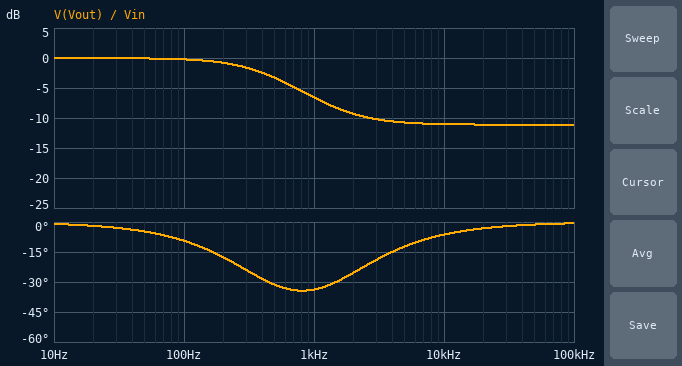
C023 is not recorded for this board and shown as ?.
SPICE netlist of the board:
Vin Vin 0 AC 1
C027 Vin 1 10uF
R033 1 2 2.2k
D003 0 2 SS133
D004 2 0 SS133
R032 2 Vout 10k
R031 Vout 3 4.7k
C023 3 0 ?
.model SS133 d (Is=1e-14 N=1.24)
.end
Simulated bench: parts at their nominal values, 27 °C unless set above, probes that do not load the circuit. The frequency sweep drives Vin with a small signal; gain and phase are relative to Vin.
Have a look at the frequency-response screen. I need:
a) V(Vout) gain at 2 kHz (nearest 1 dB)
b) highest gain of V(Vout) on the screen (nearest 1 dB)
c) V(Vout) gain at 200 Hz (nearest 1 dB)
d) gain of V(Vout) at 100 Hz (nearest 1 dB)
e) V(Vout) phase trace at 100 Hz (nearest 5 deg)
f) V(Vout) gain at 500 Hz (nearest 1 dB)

-9 dB
0 dB
-1 dB
0 dB
-10 deg
-3 dB
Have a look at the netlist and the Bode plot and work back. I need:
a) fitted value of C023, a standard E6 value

22 nF
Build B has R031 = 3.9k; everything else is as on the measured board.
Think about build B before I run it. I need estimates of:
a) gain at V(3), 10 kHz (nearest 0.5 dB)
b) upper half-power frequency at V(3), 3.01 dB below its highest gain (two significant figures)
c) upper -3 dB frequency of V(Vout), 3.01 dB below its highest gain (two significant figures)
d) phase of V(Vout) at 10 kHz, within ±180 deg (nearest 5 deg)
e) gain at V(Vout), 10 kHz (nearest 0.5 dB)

-27.0 dB
450 Hz
480 Hz
-10 deg
-12.0 dB
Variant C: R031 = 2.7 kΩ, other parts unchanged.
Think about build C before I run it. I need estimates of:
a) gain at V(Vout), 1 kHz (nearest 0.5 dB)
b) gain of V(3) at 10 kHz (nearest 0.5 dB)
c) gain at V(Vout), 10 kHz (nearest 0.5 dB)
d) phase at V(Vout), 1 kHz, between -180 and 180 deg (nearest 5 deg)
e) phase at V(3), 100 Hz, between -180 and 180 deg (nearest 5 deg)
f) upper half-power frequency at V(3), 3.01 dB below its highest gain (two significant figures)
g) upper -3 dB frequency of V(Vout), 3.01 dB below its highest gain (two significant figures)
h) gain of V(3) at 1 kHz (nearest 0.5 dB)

-6.5 dB
-26.5 dB
-14.5 dB
-45 deg
-10 deg
490 Hz
500 Hz
-7.0 dB
